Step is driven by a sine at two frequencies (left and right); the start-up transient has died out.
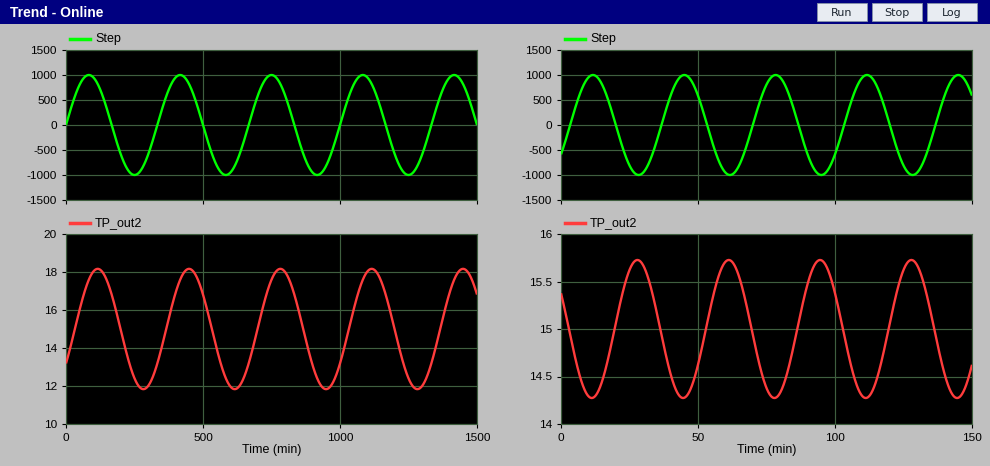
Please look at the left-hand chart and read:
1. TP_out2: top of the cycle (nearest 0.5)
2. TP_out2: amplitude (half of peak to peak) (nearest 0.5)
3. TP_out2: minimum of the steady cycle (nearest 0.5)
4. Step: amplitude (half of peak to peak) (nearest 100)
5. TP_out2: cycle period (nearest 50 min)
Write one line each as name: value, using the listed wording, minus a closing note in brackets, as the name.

TP_out2: top of the cycle: 18.0
TP_out2: amplitude (half of peak to peak): 3.0
TP_out2: minimum of the steady cycle: 12.0
Step: amplitude (half of peak to peak): 1000
TP_out2: cycle period: 350 min
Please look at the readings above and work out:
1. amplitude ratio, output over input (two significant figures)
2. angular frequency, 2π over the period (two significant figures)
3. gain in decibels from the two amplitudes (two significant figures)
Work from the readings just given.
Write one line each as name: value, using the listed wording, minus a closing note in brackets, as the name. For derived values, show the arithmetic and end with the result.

amplitude ratio, output over input: 3 / 1000 = 0.0030
angular frequency, 2π over the period: 2π / 350 = 0.018 rad/min
gain in decibels from the two amplitudes: 20 log10(3 / 1000) = -50 dB
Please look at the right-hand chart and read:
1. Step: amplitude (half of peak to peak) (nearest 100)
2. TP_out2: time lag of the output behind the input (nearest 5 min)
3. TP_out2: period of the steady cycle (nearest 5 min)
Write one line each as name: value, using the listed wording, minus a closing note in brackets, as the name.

Step: amplitude (half of peak to peak): 1000
TP_out2: time lag of the output behind the input: 15 min
TP_out2: period of the steady cycle: 35 min
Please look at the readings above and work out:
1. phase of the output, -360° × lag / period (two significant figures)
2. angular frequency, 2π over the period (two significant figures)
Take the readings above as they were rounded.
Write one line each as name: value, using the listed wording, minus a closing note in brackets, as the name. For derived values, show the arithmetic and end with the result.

phase of the output, -360° × lag / period: -360 × 15 / 35 = -150°
angular frequency, 2π over the period: 2π / 35 = 0.18 rad/min
